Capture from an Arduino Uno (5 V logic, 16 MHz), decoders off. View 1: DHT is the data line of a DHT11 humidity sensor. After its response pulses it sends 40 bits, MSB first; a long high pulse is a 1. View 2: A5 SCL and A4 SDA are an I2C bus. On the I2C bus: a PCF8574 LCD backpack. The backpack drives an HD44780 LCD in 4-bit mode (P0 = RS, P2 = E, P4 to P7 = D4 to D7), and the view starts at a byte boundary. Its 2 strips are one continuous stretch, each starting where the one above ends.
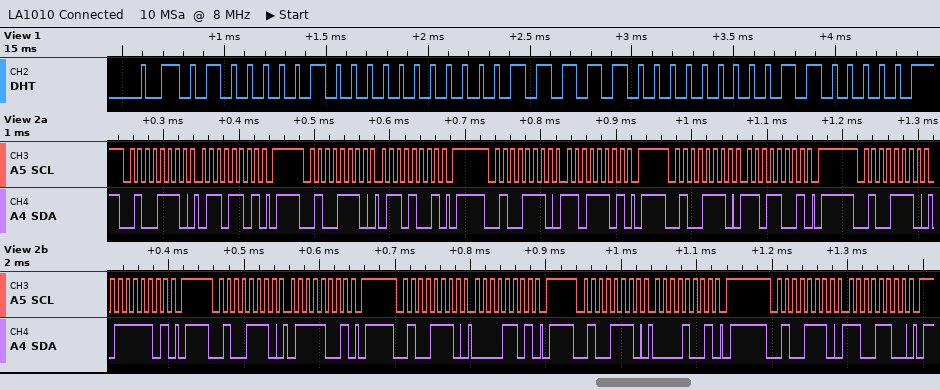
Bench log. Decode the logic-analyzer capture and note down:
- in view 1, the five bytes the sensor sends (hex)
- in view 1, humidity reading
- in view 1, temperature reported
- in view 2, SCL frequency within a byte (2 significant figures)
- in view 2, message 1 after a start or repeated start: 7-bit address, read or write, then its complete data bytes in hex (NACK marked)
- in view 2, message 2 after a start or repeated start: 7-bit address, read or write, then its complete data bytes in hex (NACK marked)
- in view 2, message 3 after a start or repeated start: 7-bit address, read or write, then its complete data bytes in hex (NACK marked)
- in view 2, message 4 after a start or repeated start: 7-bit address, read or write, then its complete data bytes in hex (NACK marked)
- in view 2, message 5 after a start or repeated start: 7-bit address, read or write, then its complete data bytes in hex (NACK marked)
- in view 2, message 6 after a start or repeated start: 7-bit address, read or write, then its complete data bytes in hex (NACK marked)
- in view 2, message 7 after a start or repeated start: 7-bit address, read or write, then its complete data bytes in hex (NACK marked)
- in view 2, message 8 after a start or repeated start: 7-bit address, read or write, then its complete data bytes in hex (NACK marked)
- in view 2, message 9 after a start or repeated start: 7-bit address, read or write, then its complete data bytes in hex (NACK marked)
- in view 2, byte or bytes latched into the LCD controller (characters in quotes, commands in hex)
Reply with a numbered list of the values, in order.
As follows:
1. 41 00 1F 00 60
2. 65 %
3. 31.0 °C
4. 100 kHz
5. 0x27 write: 6D
6. 0x27 write: 69
7. 0x27 write: DD
8. 0x27 write: D9
9. 0x27 write: 7D
10. 0x27 write: 79
11. 0x27 write: 0D
12. 0x27 write: 09
13. 0x27 write: CC
14. 'm' 'p'
